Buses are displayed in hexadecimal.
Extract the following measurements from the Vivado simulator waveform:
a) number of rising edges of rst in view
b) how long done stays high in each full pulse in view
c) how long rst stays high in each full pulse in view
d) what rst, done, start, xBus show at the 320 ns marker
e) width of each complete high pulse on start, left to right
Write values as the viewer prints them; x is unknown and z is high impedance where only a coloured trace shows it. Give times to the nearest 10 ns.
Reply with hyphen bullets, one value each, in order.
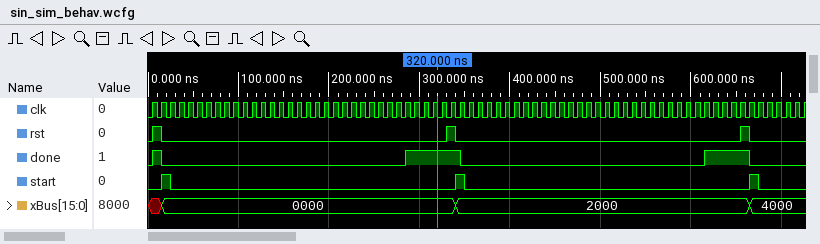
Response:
- 3
- 10 ns, 60 ns, 50 ns
- 10 ns, 10 ns, 10 ns
- rst=0, done=1, start=0, xBus=0000
- 10 ns, 10 ns, 10 ns
